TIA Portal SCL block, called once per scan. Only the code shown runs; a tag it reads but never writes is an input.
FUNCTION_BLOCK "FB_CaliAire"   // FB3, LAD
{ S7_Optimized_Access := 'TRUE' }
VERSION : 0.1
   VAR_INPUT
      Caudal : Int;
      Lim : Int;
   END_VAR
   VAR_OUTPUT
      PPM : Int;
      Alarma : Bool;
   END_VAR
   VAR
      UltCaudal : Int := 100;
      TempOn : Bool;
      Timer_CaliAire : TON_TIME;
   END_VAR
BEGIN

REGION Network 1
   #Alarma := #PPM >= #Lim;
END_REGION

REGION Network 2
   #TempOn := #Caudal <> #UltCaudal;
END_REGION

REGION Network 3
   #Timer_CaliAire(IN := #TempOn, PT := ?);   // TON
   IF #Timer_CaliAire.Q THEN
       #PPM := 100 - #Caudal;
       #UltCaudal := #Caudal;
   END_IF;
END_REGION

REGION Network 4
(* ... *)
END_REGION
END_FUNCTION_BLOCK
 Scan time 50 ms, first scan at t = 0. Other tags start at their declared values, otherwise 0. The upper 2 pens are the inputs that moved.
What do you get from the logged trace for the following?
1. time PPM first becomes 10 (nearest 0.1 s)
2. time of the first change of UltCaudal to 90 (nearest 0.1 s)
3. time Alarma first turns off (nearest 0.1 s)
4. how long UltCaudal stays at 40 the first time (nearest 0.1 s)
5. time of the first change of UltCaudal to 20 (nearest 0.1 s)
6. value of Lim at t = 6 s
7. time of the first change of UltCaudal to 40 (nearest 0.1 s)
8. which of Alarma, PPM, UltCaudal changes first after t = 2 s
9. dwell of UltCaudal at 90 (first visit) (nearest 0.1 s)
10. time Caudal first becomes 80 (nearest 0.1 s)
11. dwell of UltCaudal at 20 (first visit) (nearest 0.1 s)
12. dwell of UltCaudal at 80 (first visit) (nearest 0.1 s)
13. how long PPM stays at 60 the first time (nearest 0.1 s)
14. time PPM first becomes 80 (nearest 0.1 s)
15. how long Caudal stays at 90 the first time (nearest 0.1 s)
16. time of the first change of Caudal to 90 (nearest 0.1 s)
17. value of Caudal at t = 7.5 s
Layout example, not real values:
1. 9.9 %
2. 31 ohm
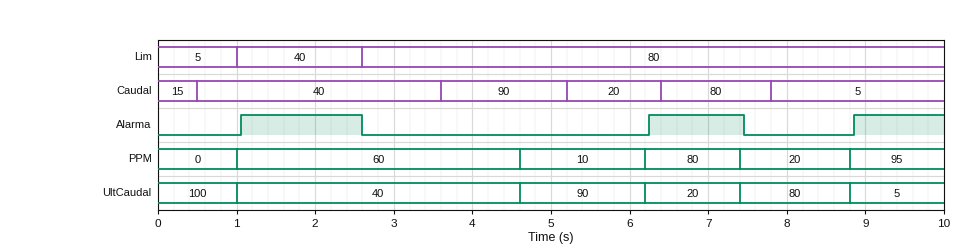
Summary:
1. 4.6 s
2. 4.6 s
3. 2.6 s
4. 3.6 s
5. 6.2 s
6. 80
7. 1.0 s
8. Alarma
9. 1.6 s
10. 6.4 s
11. 1.2 s
12. 1.4 s
13. 3.6 s
14. 6.2 s
15. 1.6 s
16. 3.6 s
17. 80
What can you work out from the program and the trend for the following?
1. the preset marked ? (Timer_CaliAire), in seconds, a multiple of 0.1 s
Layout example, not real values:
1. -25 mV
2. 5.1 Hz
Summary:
1. 1.0 s
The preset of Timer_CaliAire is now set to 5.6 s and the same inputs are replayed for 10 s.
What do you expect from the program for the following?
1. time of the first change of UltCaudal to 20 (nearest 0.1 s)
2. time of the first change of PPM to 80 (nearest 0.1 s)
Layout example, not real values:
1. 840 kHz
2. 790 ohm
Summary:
1. 5.6 s
2. 5.6 s
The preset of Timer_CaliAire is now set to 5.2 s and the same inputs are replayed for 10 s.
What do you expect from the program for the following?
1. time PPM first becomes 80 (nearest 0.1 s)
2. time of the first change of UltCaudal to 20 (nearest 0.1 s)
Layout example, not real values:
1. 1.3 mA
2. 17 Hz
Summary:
1. 5.2 s
2. 5.2 s
